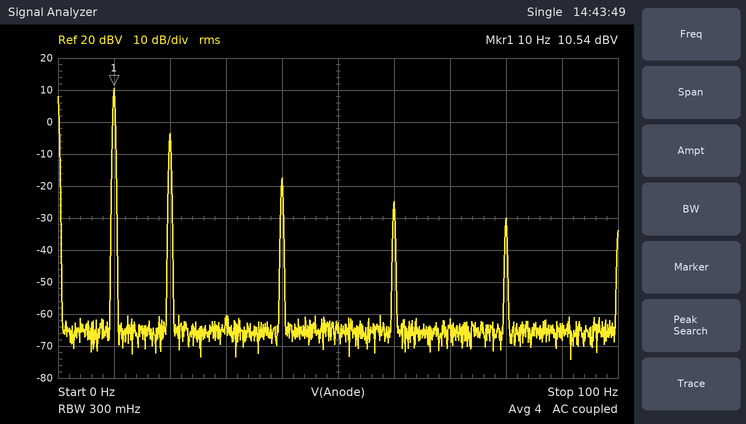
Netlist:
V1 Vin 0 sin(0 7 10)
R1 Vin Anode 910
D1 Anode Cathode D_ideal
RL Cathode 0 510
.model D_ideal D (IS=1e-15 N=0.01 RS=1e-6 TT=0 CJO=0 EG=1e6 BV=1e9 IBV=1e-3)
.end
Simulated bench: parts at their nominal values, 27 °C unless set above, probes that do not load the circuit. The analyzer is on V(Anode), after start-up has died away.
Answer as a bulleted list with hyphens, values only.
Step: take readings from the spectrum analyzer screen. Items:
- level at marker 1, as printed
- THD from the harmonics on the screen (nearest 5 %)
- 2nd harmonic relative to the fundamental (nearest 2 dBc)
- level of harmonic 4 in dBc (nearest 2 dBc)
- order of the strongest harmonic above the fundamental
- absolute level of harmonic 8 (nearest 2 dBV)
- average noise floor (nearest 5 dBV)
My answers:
- 10.54 dBV
- 20 %
- -14 dBc
- -28 dBc
- 2
- -30 dBV
- -65 dBV
